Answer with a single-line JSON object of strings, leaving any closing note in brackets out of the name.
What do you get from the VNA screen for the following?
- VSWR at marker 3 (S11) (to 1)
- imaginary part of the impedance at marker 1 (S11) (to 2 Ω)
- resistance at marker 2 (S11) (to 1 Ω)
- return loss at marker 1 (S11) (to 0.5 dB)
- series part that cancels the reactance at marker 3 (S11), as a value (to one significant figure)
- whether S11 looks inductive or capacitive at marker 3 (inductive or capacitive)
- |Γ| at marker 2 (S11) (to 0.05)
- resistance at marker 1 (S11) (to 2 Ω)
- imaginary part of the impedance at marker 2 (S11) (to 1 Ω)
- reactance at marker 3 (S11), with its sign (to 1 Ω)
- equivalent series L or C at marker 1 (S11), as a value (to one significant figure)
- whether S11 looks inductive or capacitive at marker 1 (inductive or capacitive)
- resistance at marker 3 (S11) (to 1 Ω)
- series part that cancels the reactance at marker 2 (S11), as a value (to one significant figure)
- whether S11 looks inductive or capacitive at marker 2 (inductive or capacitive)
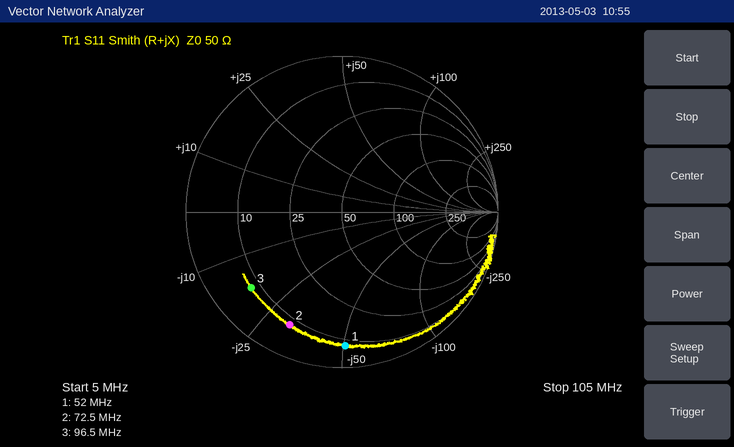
{"VSWR at marker 3 (S11)": "7", "imaginary part of the impedance at marker 1 (S11)": "-50 Ω", "resistance at marker 2 (S11)": "8 Ω", "return loss at marker 1 (S11)": "1.5 dB", "series part that cancels the reactance at marker 3 (S11), as a value": "30 nH", "whether S11 looks inductive or capacitive at marker 3": "capacitive", "|Γ| at marker 2 (S11)": "0.80", "resistance at marker 1 (S11)": "8 Ω", "imaginary part of the impedance at marker 2 (S11)": "-31 Ω", "reactance at marker 3 (S11), with its sign": "-18 Ω", "equivalent series L or C at marker 1 (S11), as a value": "60 pF", "whether S11 looks inductive or capacitive at marker 1": "capacitive", "resistance at marker 3 (S11)": "8 Ω", "series part that cancels the reactance at marker 2 (S11), as a value": "70 nH", "whether S11 looks inductive or capacitive at marker 2": "capacitive"}
